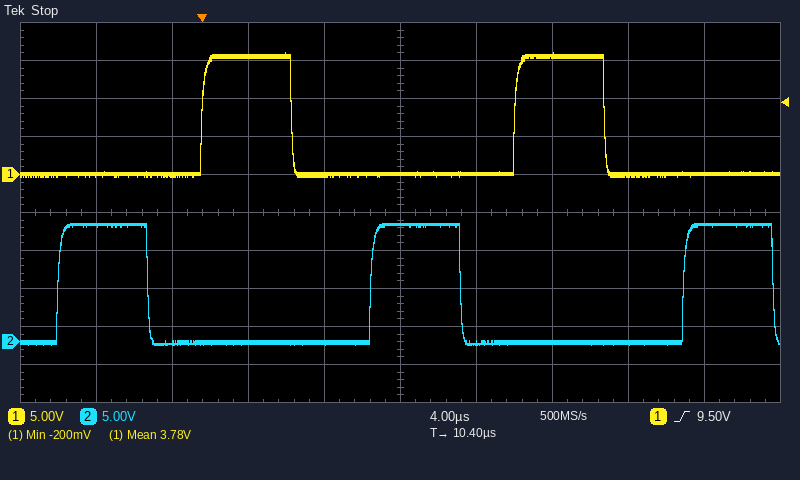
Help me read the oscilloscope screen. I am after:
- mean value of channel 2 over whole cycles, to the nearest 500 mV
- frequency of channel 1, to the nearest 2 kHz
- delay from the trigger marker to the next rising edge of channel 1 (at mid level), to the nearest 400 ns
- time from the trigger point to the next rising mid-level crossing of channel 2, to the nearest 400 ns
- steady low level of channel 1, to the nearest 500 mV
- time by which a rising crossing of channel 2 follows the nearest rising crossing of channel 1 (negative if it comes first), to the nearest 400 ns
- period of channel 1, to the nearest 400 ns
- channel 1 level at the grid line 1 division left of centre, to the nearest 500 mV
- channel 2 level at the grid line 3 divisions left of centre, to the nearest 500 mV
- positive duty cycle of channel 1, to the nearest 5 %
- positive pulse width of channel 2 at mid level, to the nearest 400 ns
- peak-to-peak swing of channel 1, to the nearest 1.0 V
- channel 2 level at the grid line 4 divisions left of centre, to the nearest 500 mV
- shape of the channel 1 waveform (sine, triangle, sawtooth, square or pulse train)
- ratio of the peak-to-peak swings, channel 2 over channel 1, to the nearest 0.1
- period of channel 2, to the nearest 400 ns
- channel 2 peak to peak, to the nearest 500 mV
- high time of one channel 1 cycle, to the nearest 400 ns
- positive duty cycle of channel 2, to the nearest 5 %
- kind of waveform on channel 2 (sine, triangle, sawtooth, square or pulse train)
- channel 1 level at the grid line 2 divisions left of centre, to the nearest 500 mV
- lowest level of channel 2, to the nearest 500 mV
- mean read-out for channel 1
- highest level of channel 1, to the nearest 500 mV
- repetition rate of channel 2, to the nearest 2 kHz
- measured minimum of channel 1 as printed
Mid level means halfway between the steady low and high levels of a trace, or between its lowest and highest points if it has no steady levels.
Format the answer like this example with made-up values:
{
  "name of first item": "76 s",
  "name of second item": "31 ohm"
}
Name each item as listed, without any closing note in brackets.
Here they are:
{
  "mean value of channel 2 over whole cycles, to the nearest 500 mV": "4.5 V",
  "frequency of channel 1, to the nearest 2 kHz": "60 kHz",
  "delay from the trigger marker to the next rising edge of channel 1 (at mid level), to the nearest 400 ns": "16.4 µs",
  "time from the trigger point to the next rising mid-level crossing of channel 2, to the nearest 400 ns": "8.8 µs",
  "steady low level of channel 1, to the nearest 500 mV": "0.0 V",
  "time by which a rising crossing of channel 2 follows the nearest rising crossing of channel 1 (negative if it comes first), to the nearest 400 ns": "-7.6 µs",
  "period of channel 1, to the nearest 400 ns": "16.4 µs",
  "channel 1 level at the grid line 1 division left of centre, to the nearest 500 mV": "0.0 V",
  "channel 2 level at the grid line 3 divisions left of centre, to the nearest 500 mV": "0.0 V",
  "positive duty cycle of channel 1, to the nearest 5 %": "30 %",
  "positive pulse width of channel 2 at mid level, to the nearest 400 ns": "4.8 µs",
  "peak-to-peak swing of channel 1, to the nearest 1.0 V": "16.0 V",
  "channel 2 level at the grid line 4 divisions left of centre, to the nearest 500 mV": "15.5 V",
  "shape of the channel 1 waveform": "pulse train",
  "ratio of the peak-to-peak swings, channel 2 over channel 1, to the nearest 0.1": "1.0",
  "period of channel 2, to the nearest 400 ns": "16.4 µs",
  "channel 2 peak to peak, to the nearest 500 mV": "16.0 V",
  "high time of one channel 1 cycle, to the nearest 400 ns": "4.8 µs",
  "positive duty cycle of channel 2, to the nearest 5 %": "30 %",
  "kind of waveform on channel 2": "pulse train",
  "channel 1 level at the grid line 2 divisions left of centre, to the nearest 500 mV": "15.5 V",
  "lowest level of channel 2, to the nearest 500 mV": "-500 mV",
  "mean read-out for channel 1": "3.78 V",
  "highest level of channel 1, to the nearest 500 mV": "16.0 V",
  "repetition rate of channel 2, to the nearest 2 kHz": "60 kHz",
  "measured minimum of channel 1 as printed": "-200 mV"
}
